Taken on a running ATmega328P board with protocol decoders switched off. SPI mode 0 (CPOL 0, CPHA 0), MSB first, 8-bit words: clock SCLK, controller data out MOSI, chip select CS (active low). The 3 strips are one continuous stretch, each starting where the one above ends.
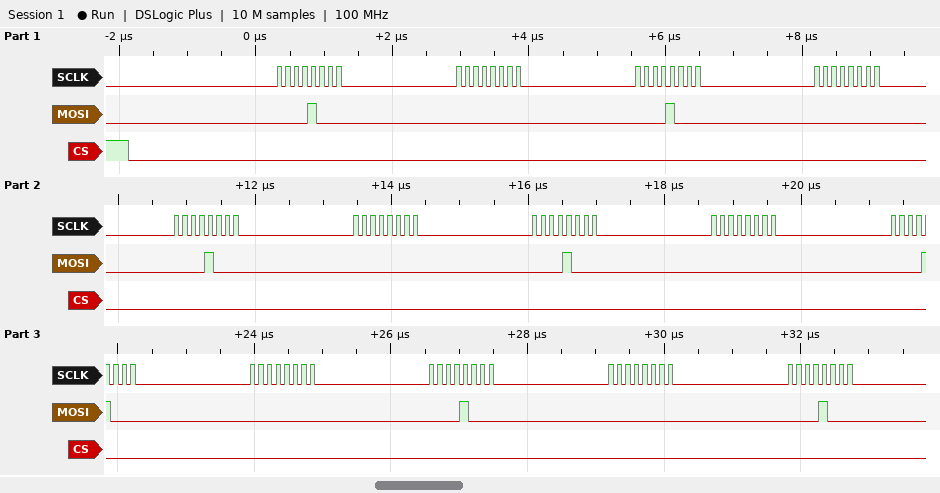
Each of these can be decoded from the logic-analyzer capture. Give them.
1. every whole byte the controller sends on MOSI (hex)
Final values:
0x08 0x00 0x08 0x00 0x08 0x00 0x08 0x00 0x08 0x00 0x08 0x00 0x08
